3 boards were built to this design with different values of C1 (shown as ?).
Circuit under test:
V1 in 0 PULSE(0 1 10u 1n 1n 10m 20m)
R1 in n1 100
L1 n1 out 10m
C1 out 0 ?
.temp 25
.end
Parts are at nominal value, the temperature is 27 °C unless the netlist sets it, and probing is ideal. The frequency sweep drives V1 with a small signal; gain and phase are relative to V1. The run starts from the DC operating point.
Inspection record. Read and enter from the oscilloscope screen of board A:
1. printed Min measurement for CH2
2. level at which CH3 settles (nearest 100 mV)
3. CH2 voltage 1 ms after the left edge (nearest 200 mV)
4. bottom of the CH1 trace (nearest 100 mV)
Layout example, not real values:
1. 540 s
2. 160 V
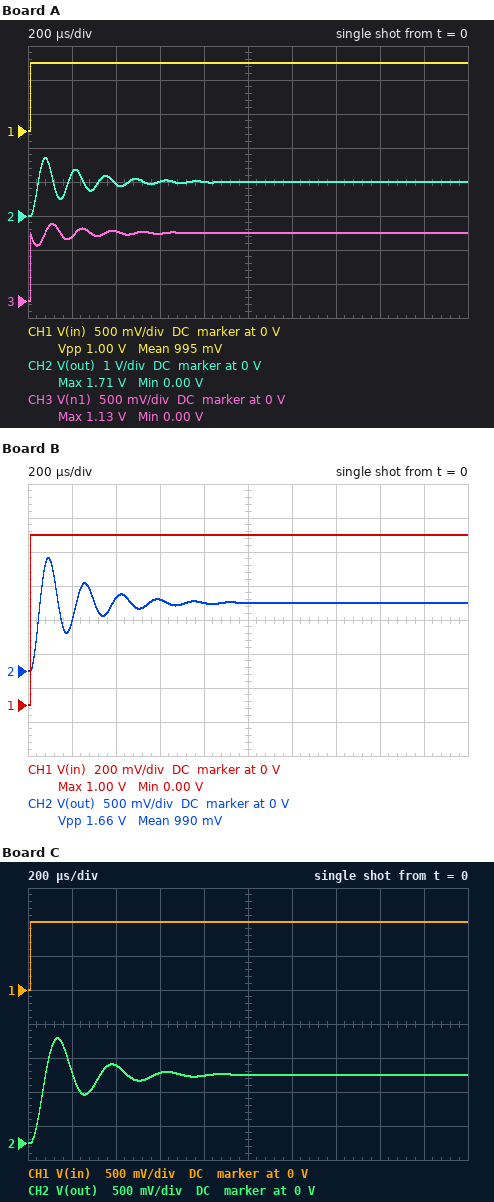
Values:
1. 0.00 V
2. 1.0 V
3. 1.0 V
4. 0 V
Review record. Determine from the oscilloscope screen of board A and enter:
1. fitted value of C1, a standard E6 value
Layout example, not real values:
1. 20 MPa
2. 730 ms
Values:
1. 47 nF
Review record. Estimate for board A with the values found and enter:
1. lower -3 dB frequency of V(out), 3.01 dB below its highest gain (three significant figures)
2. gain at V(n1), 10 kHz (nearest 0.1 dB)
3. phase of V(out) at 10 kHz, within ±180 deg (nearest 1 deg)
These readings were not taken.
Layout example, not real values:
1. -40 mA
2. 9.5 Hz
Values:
1. 6.40 kHz
2. -0.5 dB
3. -161 deg
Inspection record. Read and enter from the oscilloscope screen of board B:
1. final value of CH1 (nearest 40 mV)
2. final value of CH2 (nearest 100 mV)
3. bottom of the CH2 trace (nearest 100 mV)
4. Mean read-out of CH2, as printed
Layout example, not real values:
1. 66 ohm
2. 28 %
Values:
1. 1.00 V
2. 1.0 V
3. 0 V
4. 990 mV
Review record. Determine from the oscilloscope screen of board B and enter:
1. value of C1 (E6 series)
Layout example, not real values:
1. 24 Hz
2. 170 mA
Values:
1. 68 nF
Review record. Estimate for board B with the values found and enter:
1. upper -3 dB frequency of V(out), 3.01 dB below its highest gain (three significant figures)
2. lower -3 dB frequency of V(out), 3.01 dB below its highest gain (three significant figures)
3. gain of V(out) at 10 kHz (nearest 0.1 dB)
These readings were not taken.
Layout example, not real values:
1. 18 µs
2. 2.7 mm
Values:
1. 6.75 kHz
2. 5.13 kHz
3. -4.8 dB
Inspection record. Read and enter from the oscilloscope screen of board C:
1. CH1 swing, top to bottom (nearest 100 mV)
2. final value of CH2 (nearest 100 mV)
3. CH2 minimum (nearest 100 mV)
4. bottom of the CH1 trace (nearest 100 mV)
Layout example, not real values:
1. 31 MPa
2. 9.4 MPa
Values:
1. 1.0 V
2. 1.0 V
3. 0 V
4. 0 V
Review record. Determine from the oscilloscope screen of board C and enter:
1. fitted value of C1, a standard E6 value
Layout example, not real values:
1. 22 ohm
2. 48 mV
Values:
1. 150 nF
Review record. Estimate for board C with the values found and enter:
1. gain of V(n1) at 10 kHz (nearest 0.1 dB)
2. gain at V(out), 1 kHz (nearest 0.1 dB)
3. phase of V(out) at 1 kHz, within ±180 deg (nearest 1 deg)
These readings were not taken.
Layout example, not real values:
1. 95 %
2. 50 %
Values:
1. -0.2 dB
2. 0.5 dB
3. -6 deg
